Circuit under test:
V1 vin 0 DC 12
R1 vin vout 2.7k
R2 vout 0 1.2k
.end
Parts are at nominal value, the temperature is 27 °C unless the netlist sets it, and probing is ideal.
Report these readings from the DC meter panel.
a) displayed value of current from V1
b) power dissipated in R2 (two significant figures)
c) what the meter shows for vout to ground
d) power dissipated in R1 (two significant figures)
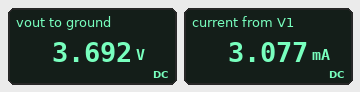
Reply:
3.077 mA
11 mW
3.692 V
26 mW
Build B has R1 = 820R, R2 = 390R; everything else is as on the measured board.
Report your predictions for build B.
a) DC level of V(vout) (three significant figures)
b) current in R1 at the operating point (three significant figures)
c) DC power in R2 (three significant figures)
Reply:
3.87 V
9.92 mA
38.4 mW
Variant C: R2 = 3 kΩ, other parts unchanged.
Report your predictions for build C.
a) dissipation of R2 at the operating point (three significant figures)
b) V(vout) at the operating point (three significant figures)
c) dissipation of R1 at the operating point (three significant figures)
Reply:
13.3 mW
6.32 V
12.0 mW
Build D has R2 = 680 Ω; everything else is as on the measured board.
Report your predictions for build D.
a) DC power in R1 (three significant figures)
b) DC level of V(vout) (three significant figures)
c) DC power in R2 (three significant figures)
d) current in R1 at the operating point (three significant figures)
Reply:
34.0 mW
2.41 V
8.57 mW
3.55 mA
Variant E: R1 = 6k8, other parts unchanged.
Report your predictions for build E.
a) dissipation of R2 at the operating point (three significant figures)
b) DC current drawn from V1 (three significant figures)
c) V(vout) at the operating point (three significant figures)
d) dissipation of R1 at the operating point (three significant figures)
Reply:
2.70 mW
1.50 mA
1.80 V
15.3 mW
